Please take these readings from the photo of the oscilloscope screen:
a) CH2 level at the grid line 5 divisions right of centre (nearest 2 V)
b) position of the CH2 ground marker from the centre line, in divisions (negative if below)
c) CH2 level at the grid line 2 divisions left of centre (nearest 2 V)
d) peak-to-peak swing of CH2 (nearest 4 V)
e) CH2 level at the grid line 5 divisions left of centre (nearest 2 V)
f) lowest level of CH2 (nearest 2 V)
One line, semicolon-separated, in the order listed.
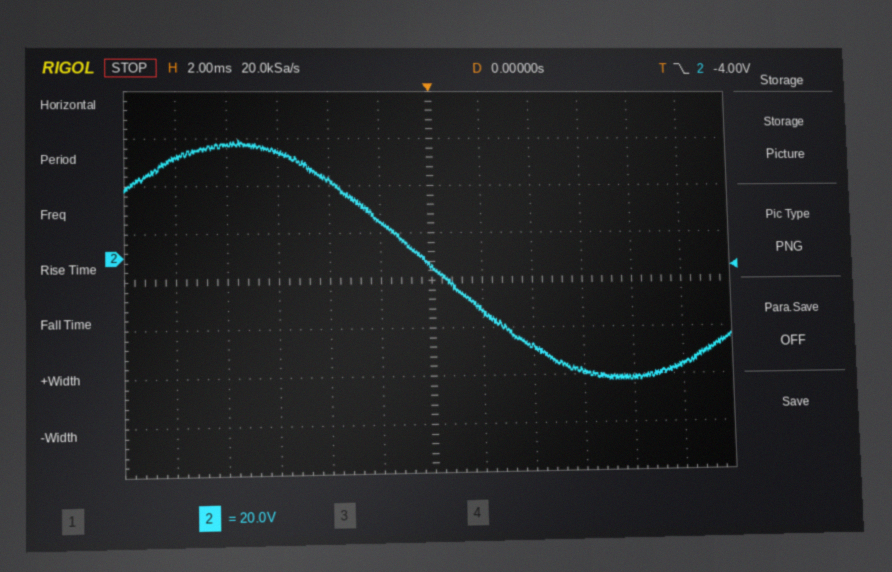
-46 V; +0.5 div; 32 V; 100 V; 42 V; -52 V
